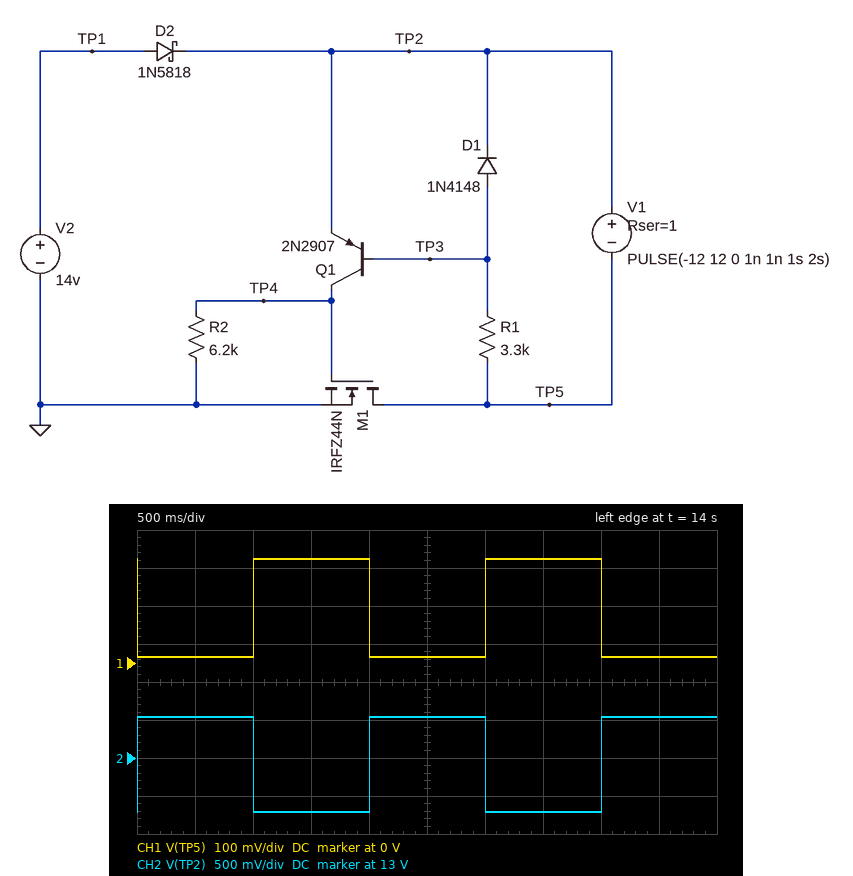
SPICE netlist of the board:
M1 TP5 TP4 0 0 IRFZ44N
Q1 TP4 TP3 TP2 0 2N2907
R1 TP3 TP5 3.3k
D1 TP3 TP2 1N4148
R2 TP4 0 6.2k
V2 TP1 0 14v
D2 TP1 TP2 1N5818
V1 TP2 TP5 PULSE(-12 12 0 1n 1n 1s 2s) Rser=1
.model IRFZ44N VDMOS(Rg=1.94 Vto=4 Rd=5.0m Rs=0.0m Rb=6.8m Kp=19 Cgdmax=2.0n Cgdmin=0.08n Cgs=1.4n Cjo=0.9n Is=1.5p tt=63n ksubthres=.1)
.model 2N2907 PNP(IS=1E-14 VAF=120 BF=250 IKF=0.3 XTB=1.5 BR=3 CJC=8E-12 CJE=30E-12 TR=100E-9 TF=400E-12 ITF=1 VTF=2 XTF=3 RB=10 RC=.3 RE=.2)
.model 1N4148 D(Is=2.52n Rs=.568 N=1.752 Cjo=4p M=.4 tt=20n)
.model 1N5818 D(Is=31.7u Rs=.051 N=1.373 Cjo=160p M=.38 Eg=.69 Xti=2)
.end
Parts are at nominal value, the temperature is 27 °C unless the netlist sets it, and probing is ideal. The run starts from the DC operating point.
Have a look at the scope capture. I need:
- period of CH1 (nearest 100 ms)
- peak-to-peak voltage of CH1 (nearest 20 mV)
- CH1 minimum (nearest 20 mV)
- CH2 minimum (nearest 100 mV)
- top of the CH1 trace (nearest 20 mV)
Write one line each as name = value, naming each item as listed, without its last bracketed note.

period of CH1 = 2.0 s
peak-to-peak voltage of CH1 = 260 mV
CH1 minimum = 20 mV
CH2 minimum = 12.3 V
top of the CH1 trace = 280 mV
